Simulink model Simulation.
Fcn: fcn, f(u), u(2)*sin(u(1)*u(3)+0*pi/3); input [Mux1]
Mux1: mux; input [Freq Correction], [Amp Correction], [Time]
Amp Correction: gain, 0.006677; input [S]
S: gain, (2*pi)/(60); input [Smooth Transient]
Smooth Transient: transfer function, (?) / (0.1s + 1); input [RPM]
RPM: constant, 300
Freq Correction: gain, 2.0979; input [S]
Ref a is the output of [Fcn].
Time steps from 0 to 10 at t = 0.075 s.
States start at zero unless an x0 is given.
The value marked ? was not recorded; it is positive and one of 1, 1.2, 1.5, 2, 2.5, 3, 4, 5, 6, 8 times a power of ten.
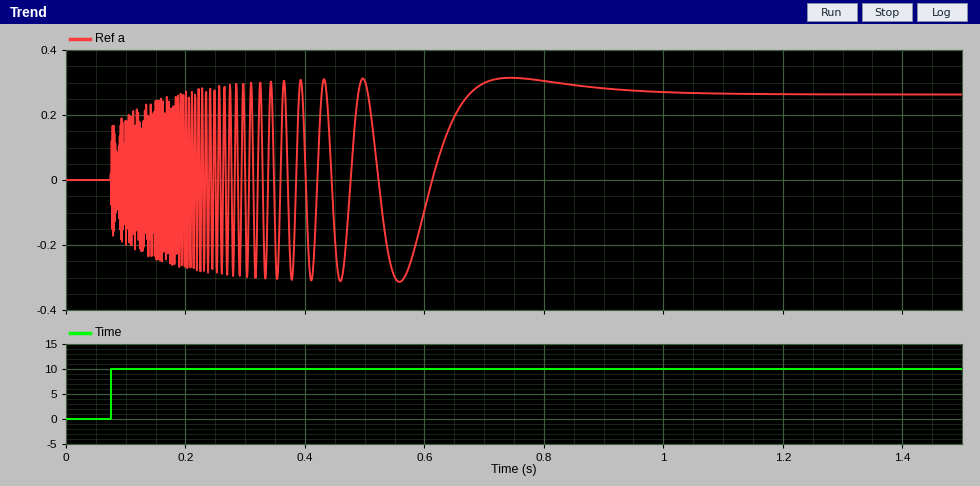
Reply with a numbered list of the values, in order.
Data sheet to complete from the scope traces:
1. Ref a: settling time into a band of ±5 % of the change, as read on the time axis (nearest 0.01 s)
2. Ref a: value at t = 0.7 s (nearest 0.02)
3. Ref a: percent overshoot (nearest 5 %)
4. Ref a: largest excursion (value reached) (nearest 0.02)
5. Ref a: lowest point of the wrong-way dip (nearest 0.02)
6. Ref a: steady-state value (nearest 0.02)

1. 0.94 s
2. 0.30
3. 20 %
4. 0.32
5. -0.32
6. 0.26
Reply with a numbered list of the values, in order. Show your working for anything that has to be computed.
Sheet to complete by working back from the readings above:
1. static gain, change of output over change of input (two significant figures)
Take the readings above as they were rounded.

1. (0.26 - 0) / (10 - 0) = 0.026
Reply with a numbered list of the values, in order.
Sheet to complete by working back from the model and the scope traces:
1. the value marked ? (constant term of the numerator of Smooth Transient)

1. 1.5
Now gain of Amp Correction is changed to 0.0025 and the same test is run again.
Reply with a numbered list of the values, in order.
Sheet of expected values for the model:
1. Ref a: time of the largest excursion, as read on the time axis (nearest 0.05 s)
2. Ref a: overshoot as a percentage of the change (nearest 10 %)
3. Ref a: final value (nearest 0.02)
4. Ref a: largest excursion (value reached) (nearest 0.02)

1. 0.75 s
2. 20 %
3. 0.10
4. 0.12
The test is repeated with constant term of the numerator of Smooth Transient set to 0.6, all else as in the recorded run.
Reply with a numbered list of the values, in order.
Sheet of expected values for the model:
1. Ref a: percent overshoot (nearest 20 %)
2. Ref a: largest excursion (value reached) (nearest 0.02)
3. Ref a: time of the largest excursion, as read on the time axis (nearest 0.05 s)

1. 160 %
2. -0.12
3. 0.60 s
